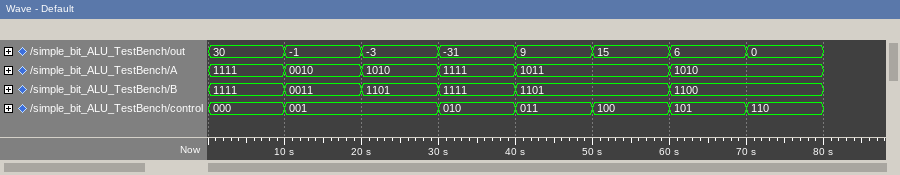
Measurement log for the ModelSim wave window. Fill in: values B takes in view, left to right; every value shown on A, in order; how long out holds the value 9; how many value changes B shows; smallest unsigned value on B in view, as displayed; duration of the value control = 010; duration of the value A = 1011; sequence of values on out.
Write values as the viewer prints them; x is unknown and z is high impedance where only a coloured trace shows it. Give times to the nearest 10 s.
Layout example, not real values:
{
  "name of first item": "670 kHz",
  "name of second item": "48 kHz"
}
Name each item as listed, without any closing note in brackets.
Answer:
{
  "values B takes in view, left to right": "1111, 0011, 1101, 1111, 1101, 1100",
  "every value shown on A, in order": "1111, 0010, 1010, 1111, 1011, 1010",
  "how long out holds the value 9": "10 s",
  "how many value changes B shows": "5",
  "smallest unsigned value on B in view, as displayed": "0011",
  "duration of the value control = 010": "10 s",
  "duration of the value A = 1011": "20 s",
  "sequence of values on out": "30, -1, -3, -31, 9, 15, 6, 0"
}
